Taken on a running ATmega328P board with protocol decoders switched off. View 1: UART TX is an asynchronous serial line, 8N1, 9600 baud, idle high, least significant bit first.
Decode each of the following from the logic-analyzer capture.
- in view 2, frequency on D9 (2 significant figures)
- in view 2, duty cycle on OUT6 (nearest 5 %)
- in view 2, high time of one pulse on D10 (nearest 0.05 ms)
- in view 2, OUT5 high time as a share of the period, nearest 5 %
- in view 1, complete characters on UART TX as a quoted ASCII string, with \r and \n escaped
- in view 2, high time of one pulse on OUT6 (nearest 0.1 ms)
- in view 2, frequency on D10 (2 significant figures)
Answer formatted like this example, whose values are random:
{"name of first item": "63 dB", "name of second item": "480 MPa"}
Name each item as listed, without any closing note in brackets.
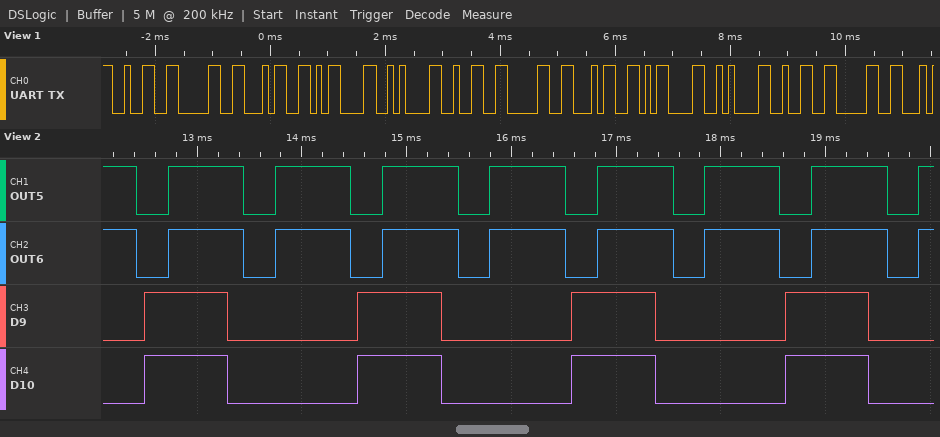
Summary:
{"in view 2, frequency on D9": "490 Hz", "in view 2, duty cycle on OUT6": "70 %", "in view 2, high time of one pulse on D10": "0.80 ms", "in view 2, OUT5 high time as a share of the period, nearest 5 %": "70 %", "in view 1, complete characters on UART TX as a quoted ASCII string, with \\r and \\n escaped": "\"204\\r\\n204\\r\\n20\"", "in view 2, high time of one pulse on OUT6": "0.7 ms", "in view 2, frequency on D10": "490 Hz"}
